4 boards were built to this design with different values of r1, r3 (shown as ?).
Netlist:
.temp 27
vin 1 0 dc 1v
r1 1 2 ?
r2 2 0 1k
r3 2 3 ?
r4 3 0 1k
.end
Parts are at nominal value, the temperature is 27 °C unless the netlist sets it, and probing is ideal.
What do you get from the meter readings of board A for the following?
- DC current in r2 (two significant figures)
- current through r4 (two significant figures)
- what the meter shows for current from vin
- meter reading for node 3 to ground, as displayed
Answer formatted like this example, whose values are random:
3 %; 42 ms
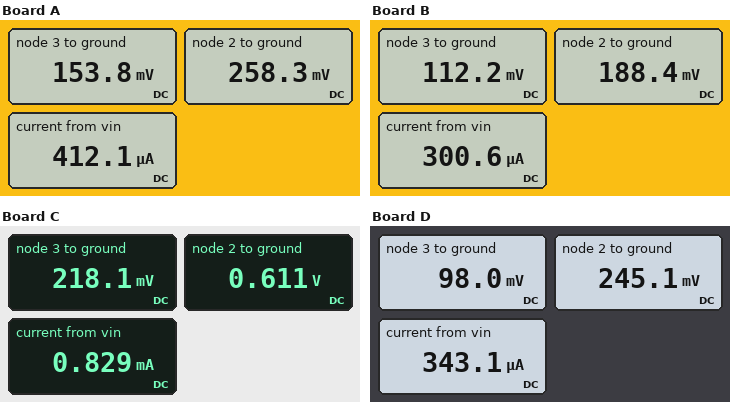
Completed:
260 µA; 150 µA; 412.1 µA; 153.8 mV
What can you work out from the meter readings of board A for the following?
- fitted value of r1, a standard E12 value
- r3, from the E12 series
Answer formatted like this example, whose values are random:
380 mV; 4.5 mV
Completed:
1.8 kΩ; 680 Ω
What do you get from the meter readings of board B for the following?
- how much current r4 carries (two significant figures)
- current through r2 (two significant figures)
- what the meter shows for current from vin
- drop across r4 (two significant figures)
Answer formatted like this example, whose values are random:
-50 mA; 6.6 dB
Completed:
110 µA; 190 µA; 300.6 µA; 110 mV
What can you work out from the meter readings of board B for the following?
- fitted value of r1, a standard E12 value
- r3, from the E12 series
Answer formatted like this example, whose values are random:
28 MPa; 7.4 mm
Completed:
2.7 kΩ; 680 Ω
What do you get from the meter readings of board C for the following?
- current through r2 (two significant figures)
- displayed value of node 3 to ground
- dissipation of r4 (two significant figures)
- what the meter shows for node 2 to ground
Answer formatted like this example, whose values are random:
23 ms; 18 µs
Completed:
610 µA; 218.1 mV; 48 µW; 0.611 V
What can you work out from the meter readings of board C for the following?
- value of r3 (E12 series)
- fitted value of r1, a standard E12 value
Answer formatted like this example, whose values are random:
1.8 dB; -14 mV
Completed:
1.8 kΩ; 470 Ω
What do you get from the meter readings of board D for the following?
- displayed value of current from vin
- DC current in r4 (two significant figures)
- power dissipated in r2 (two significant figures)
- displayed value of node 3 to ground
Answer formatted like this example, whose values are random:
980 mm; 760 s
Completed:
343.1 µA; 98 µA; 60 µW; 98.0 mV
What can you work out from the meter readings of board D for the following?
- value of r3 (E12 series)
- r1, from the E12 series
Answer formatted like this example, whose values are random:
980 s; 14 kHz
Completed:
1.5 kΩ; 2.2 kΩ
